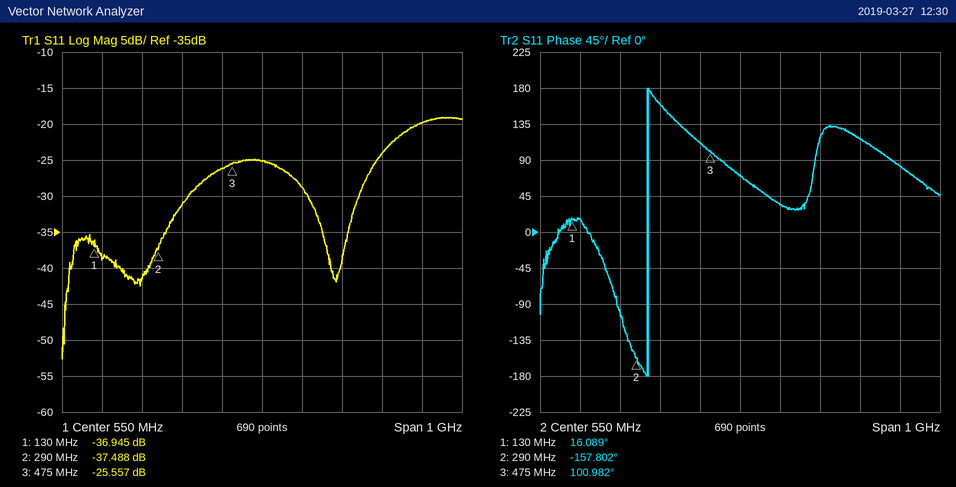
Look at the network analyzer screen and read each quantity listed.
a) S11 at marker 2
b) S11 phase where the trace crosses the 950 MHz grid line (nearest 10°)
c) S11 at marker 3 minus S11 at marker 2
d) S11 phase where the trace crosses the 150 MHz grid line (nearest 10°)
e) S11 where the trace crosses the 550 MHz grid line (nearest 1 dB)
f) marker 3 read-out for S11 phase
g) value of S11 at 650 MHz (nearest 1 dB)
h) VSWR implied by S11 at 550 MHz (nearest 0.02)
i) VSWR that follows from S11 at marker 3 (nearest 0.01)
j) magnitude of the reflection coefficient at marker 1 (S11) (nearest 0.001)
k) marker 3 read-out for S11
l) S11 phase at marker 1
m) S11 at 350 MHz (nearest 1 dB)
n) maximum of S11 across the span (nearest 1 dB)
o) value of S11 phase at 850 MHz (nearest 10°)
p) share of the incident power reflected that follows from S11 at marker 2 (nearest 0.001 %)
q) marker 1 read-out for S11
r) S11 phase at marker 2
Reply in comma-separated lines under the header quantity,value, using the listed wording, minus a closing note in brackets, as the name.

quantity,value
S11 at marker 2,-37.488 dB
S11 phase where the trace crosses the 950 MHz grid line,80°
S11 at marker 3 minus S11 at marker 2,11.931 dB
S11 phase where the trace crosses the 150 MHz grid line,20°
S11 where the trace crosses the 550 MHz grid line,-25 dB
marker 3 read-out for S11 phase,100.982°
value of S11 at 650 MHz,-29 dB
VSWR implied by S11 at 550 MHz,1.12
VSWR that follows from S11 at marker 3,1.11
magnitude of the reflection coefficient at marker 1 (S11),0.014
marker 3 read-out for S11,-25.557 dB
S11 phase at marker 1,16.089°
S11 at 350 MHz,-31 dB
maximum of S11 across the span,-19 dB
value of S11 phase at 850 MHz,120°
share of the incident power reflected that follows from S11 at marker 2,0.018 %
marker 1 read-out for S11,-36.945 dB
S11 phase at marker 2,-157.802°
